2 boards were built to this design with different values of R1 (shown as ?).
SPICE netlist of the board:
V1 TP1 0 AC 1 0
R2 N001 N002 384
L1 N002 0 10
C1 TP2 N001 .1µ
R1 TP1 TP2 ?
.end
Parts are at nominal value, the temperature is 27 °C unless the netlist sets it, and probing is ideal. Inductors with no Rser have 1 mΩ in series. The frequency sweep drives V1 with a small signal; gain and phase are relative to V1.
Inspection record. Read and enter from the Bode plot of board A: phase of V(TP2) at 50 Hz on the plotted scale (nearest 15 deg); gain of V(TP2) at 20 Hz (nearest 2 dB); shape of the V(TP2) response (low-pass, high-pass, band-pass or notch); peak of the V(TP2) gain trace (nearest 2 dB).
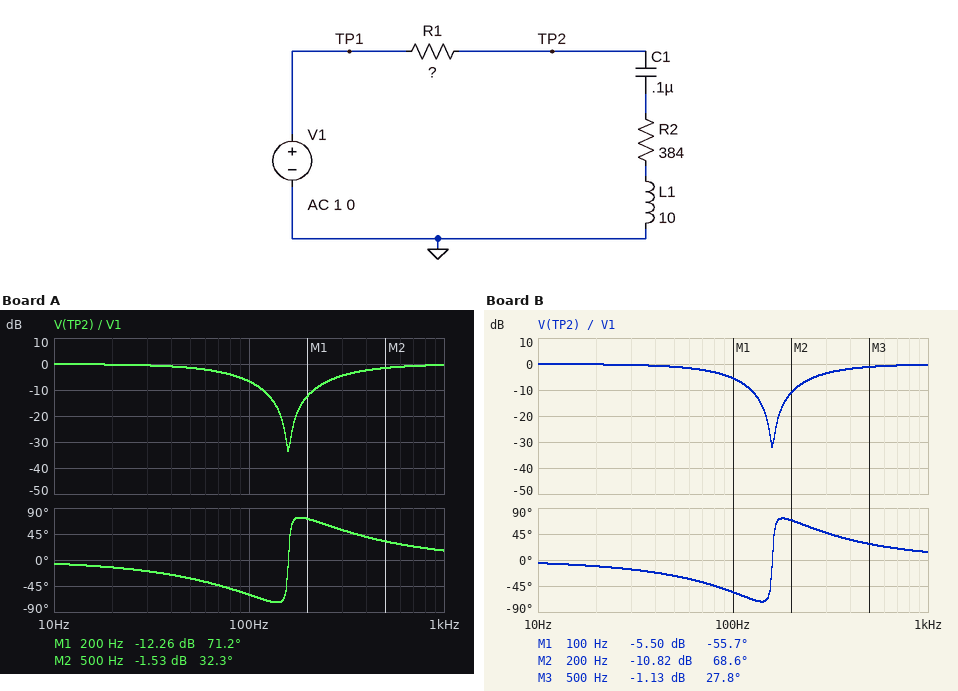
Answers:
-30 deg
0 dB
notch
0 dB
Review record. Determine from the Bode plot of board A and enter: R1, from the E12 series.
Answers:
18 kΩ
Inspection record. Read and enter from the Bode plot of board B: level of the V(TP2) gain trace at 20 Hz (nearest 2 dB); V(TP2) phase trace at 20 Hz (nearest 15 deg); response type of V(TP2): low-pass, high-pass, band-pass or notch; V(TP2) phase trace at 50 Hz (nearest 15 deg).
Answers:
0 dB
-15 deg
notch
-30 deg
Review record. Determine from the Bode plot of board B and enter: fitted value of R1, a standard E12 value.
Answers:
15 kΩ
